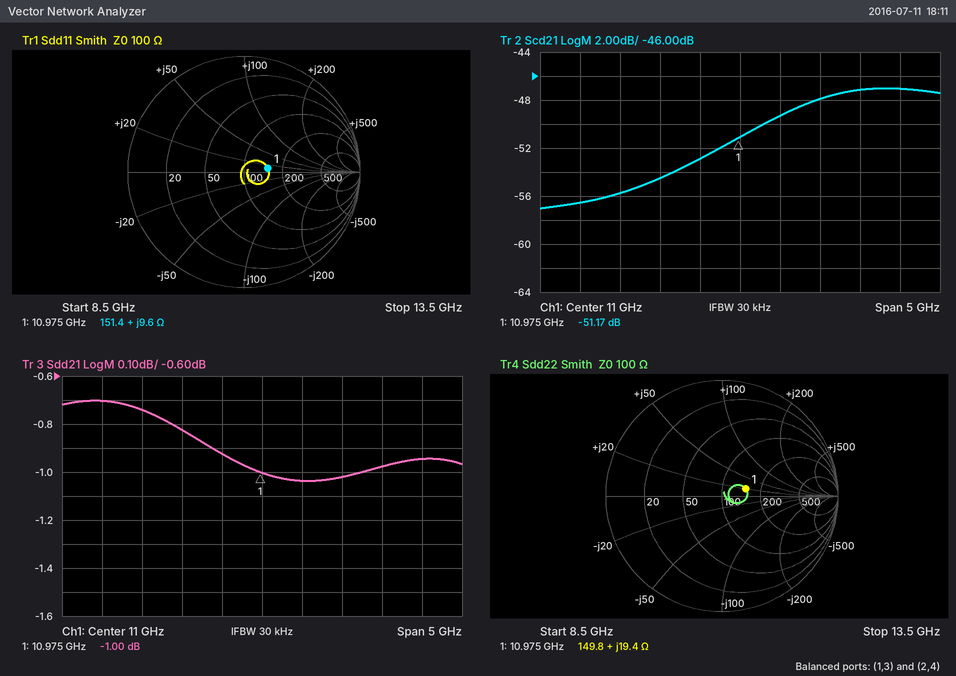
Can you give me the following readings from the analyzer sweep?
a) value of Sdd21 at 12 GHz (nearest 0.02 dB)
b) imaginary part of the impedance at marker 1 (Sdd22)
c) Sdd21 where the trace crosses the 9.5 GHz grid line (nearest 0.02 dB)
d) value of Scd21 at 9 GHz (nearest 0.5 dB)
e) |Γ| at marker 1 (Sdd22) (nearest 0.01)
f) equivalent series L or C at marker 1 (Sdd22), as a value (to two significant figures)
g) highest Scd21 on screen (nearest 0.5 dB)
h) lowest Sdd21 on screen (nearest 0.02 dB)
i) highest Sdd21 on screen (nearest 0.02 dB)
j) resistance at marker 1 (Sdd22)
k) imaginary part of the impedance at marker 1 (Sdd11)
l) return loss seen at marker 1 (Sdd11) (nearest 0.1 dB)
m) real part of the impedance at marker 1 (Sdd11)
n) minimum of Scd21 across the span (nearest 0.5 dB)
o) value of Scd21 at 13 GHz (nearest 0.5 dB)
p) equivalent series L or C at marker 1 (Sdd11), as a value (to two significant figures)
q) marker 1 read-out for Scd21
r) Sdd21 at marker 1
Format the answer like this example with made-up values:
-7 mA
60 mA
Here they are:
-1.02 dB
+19.4 Ω
-0.74 dB
-56.5 dB
0.21
280 pH
-47.0 dB
-1.04 dB
-0.70 dB
149.8 Ω
+9.6 Ω
13.6 dB
151.4 Ω
-57.0 dB
-47.0 dB
140 pH
-51.17 dB
-1.00 dB
